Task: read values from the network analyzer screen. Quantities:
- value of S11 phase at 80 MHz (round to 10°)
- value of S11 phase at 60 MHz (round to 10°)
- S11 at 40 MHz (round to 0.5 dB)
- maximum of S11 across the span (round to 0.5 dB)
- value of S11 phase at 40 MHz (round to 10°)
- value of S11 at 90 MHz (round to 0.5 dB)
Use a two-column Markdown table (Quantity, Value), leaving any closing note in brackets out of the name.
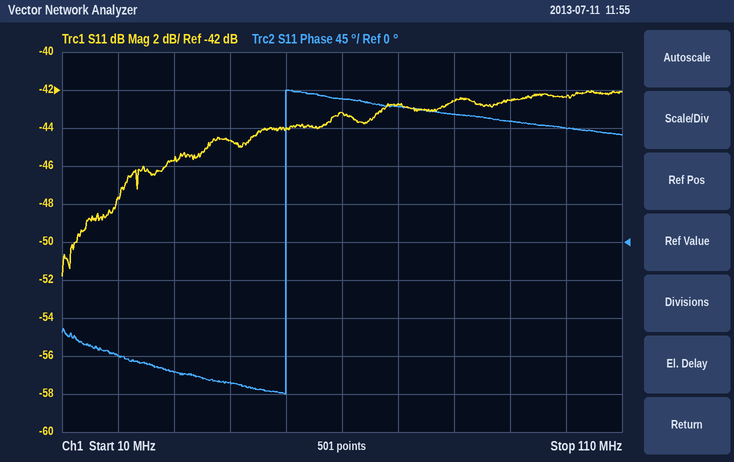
| Quantity | Value |
|---|---|
| value of S11 phase at 80 MHz | 150° |
| value of S11 phase at 60 MHz | 170° |
| S11 at 40 MHz | -44.5 dB |
| maximum of S11 across the span | -42.0 dB |
| value of S11 phase at 40 MHz | -170° |
| value of S11 at 90 MHz | -42.5 dB |
